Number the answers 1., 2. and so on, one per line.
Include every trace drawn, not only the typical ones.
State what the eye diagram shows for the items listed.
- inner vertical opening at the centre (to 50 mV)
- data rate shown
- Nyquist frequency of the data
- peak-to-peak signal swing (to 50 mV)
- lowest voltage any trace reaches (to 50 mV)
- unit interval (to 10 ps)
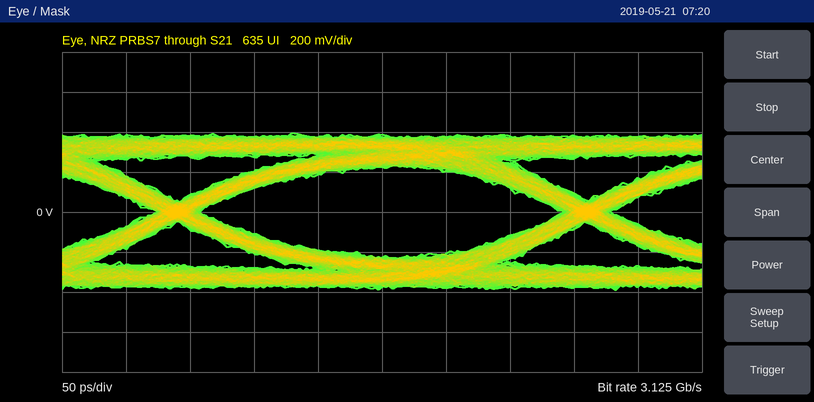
1. 450 mV
2. 3.125 Gb/s
3. 1.5625 GHz
4. 800 mV
5. -400 mV
6. 320 ps
